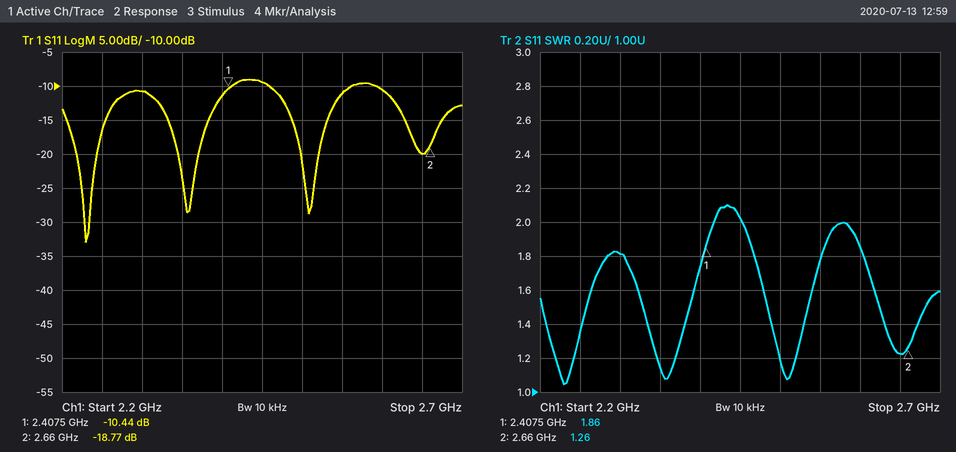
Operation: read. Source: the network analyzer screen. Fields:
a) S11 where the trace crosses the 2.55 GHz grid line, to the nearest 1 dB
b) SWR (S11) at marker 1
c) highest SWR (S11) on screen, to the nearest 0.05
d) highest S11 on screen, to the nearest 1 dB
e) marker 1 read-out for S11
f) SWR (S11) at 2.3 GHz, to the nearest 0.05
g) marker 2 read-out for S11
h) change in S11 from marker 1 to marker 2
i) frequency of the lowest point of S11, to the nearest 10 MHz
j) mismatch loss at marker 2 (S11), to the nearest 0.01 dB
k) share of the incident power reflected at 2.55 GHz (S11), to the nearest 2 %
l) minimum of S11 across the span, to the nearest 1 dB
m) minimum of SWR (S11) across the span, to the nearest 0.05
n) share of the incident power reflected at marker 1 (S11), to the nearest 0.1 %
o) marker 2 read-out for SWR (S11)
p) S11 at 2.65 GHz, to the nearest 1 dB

-11 dB
1.86
2.10
-9 dB
-10.44 dB
1.80
-18.77 dB
-8.33 dB
2.23 GHz
0.06 dB
8 %
-33 dB
1.05
9.0 %
1.26
-20 dB
